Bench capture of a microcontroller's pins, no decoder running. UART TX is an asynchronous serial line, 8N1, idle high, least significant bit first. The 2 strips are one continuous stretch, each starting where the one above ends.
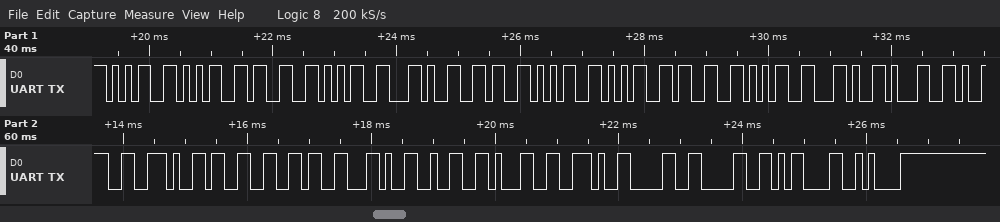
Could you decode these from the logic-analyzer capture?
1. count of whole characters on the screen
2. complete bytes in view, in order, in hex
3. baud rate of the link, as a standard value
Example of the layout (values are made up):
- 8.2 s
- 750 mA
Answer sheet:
- 24
- 35 35 33 35 2C 36 35 35 33 35 2C 31 39 2E 33 36 2C 32 31 2E 30 30 0D 0A
- 9600 baud
